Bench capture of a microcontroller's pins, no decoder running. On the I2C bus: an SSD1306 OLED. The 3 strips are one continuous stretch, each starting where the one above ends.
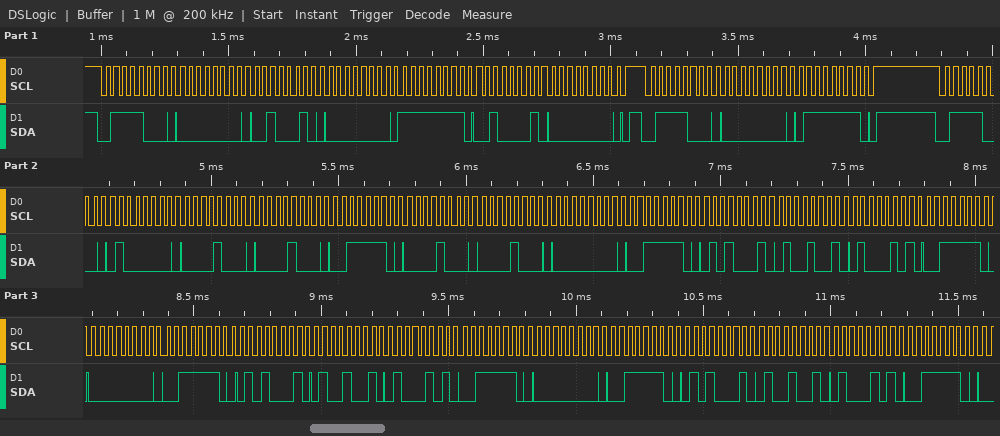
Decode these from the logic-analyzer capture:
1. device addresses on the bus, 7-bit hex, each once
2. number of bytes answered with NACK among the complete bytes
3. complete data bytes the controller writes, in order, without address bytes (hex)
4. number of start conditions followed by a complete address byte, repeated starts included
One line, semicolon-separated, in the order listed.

0x3C; 0; 00 22 00 FF 21 00 00 7F 40 08 08 3E 08 08 00 3E 51 49 45 3E 00 3E 51 49 45 3E 00 3E 51 49 45 3E; 3
